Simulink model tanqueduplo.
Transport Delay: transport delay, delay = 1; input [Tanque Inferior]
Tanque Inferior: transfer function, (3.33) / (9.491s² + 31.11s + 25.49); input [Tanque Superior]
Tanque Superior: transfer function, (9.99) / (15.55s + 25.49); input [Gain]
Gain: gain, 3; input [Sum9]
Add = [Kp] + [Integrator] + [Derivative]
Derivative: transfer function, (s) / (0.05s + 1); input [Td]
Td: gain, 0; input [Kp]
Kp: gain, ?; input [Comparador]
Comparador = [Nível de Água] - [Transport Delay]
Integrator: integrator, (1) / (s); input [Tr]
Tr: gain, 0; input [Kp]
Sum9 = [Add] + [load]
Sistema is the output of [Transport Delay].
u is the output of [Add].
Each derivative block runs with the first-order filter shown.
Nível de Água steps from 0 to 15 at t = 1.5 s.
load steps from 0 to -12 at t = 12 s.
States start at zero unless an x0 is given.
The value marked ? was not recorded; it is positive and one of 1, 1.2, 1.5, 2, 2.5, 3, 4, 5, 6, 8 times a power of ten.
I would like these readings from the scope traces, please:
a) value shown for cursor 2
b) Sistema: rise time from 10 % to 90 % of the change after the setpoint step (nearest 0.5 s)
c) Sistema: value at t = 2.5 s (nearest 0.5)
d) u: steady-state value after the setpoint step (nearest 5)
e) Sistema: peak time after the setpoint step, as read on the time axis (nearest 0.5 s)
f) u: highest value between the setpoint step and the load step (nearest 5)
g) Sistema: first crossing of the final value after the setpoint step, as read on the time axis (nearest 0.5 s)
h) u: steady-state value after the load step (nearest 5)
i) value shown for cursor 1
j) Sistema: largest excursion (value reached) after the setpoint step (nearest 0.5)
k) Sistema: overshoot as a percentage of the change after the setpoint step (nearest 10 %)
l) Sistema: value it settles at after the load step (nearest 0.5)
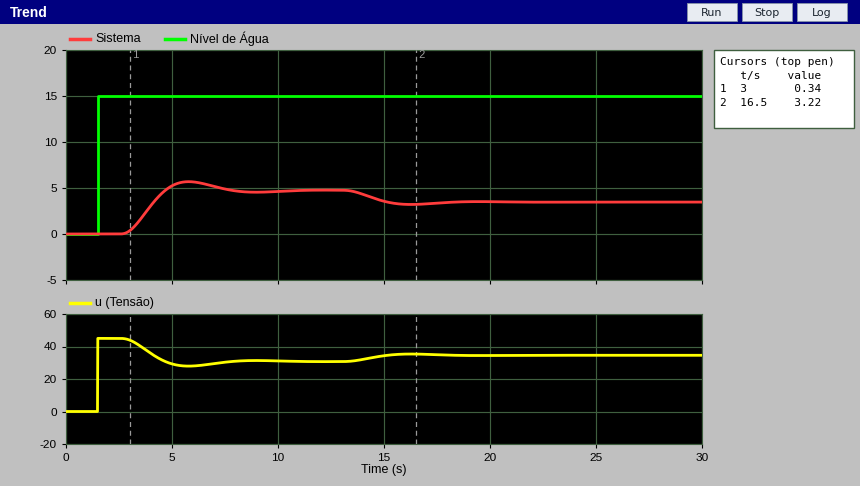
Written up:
3.22
1.5 s
0.0
30
6.0 s
45
4.5 s
35
0.34
5.5
20 %
3.5
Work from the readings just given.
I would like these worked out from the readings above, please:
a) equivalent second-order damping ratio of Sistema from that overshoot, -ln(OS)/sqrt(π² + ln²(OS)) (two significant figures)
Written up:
0.46
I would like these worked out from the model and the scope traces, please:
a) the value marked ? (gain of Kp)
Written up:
3
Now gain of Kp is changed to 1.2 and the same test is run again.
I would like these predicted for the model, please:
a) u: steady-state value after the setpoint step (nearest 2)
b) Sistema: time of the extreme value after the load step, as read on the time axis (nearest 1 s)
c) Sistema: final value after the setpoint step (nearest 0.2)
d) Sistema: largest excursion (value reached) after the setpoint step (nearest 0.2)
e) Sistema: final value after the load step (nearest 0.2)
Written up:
16
17 s
2.4
2.4
0.8
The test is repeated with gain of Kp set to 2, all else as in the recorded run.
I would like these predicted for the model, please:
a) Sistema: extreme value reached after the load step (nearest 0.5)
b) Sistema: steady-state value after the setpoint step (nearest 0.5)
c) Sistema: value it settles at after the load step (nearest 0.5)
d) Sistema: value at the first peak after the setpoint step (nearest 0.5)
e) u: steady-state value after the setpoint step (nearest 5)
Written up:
2.0
3.5
2.0
4.0
25
